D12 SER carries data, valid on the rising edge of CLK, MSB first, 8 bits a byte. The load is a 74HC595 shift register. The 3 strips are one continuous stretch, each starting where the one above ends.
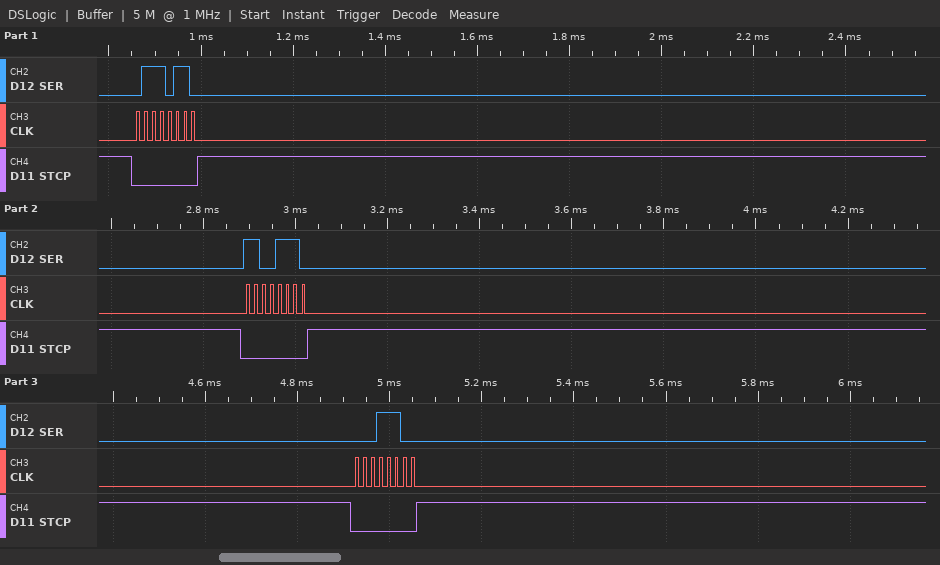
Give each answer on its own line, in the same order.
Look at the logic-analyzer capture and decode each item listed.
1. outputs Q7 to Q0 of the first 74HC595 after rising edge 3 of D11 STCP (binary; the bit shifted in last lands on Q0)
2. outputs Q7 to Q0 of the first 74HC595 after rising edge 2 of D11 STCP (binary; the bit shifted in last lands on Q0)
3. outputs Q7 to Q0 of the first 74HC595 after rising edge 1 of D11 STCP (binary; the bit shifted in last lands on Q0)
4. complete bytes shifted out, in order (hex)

00011100
11001110
01110110
76 CE 1C
